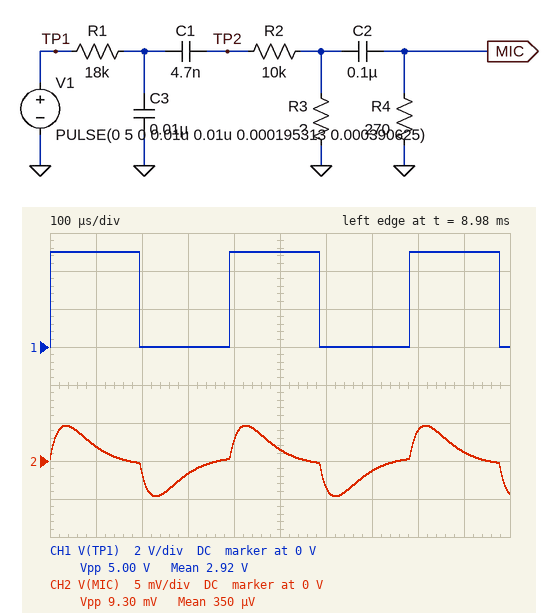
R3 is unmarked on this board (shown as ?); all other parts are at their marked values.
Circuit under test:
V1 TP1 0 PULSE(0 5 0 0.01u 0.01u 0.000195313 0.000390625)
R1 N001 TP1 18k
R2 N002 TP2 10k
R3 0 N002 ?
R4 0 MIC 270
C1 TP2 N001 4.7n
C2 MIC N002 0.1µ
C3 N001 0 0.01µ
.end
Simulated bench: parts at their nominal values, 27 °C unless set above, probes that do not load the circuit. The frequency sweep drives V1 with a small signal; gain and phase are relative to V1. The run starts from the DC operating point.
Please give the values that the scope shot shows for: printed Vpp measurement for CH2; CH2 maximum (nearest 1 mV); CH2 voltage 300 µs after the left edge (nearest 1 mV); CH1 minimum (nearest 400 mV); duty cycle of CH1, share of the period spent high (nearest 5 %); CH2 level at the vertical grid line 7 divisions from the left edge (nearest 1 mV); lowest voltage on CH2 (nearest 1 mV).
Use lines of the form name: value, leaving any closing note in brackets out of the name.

printed Vpp measurement for CH2: 9.30 mV
CH2 maximum: 5 mV
CH2 voltage 300 µs after the left edge: -2 mV
CH1 minimum: 0 V
duty cycle of CH1, share of the period spent high: 50 %
CH2 level at the vertical grid line 7 divisions from the left edge: -1 mV
lowest voltage on CH2: -5 mV
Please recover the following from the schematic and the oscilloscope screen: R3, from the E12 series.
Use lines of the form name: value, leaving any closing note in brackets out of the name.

R3, from the E12 series: 220 Ω
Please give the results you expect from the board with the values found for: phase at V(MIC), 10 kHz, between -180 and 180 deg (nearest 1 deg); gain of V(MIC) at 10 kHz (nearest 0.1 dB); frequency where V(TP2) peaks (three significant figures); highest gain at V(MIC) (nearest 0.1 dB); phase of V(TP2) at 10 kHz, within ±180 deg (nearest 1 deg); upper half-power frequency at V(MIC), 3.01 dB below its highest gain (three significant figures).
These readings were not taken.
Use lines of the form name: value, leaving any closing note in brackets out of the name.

phase at V(MIC), 10 kHz, between -180 and 180 deg: -41 deg
gain of V(MIC) at 10 kHz: -61.0 dB
frequency where V(TP2) peaks: 1.69 kHz
highest gain at V(MIC): -58.2 dB
phase of V(TP2) at 10 kHz, within ±180 deg: -59 deg
upper half-power frequency at V(MIC), 3.01 dB below its highest gain: 10.3 kHz
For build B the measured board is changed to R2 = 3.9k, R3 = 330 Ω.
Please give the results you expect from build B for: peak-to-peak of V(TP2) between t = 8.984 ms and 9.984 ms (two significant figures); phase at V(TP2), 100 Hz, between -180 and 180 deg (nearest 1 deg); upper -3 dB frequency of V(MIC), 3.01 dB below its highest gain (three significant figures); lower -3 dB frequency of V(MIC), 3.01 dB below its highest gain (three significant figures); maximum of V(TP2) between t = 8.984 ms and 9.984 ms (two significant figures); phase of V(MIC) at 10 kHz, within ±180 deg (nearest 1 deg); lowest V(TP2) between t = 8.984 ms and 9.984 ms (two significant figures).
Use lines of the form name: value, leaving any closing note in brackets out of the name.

peak-to-peak of V(TP2) between t = 8.984 ms and 9.984 ms: 400 mV
phase at V(TP2), 100 Hz, between -180 and 180 deg: 80 deg
upper -3 dB frequency of V(MIC), 3.01 dB below its highest gain: 17.4 kHz
lower -3 dB frequency of V(MIC), 3.01 dB below its highest gain: 2.05 kHz
maximum of V(TP2) between t = 8.984 ms and 9.984 ms: 200 mV
phase of V(MIC) at 10 kHz, within ±180 deg: -20 deg
lowest V(TP2) between t = 8.984 ms and 9.984 ms: -200 mV
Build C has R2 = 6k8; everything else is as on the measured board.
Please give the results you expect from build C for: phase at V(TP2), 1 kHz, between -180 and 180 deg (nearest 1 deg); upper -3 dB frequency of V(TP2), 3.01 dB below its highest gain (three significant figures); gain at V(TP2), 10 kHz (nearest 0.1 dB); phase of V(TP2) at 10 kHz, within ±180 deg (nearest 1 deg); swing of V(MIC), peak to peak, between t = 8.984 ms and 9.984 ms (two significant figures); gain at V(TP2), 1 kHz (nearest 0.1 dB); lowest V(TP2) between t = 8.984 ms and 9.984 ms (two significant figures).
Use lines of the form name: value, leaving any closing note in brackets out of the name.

phase at V(TP2), 1 kHz, between -180 and 180 deg: 22 deg
upper -3 dB frequency of V(TP2), 3.01 dB below its highest gain: 8.44 kHz
gain at V(TP2), 10 kHz: -23.0 dB
phase of V(TP2) at 10 kHz, within ±180 deg: -50 deg
swing of V(MIC), peak to peak, between t = 8.984 ms and 9.984 ms: 11 mV
gain at V(TP2), 1 kHz: -19.8 dB
lowest V(TP2) between t = 8.984 ms and 9.984 ms: -310 mV
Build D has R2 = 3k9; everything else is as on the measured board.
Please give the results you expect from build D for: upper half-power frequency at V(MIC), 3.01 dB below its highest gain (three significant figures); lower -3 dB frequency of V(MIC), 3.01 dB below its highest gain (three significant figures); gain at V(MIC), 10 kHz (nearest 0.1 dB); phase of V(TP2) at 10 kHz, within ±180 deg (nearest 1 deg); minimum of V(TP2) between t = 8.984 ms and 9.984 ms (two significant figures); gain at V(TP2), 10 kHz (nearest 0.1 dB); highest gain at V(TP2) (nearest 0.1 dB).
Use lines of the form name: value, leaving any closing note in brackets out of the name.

upper half-power frequency at V(MIC), 3.01 dB below its highest gain: 18.4 kHz
lower -3 dB frequency of V(MIC), 3.01 dB below its highest gain: 2.35 kHz
gain at V(MIC), 10 kHz: -56.1 dB
phase of V(TP2) at 10 kHz, within ±180 deg: -35 deg
minimum of V(TP2) between t = 8.984 ms and 9.984 ms: -200 mV
gain at V(TP2), 10 kHz: -25.3 dB
highest gain at V(TP2): -23.4 dB
